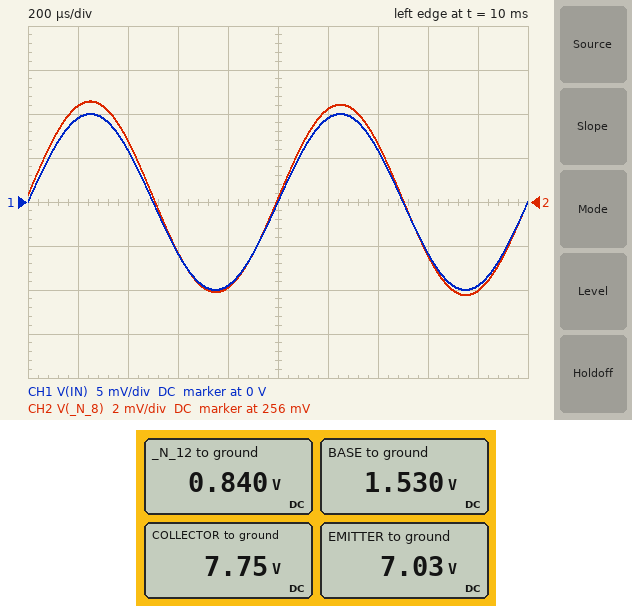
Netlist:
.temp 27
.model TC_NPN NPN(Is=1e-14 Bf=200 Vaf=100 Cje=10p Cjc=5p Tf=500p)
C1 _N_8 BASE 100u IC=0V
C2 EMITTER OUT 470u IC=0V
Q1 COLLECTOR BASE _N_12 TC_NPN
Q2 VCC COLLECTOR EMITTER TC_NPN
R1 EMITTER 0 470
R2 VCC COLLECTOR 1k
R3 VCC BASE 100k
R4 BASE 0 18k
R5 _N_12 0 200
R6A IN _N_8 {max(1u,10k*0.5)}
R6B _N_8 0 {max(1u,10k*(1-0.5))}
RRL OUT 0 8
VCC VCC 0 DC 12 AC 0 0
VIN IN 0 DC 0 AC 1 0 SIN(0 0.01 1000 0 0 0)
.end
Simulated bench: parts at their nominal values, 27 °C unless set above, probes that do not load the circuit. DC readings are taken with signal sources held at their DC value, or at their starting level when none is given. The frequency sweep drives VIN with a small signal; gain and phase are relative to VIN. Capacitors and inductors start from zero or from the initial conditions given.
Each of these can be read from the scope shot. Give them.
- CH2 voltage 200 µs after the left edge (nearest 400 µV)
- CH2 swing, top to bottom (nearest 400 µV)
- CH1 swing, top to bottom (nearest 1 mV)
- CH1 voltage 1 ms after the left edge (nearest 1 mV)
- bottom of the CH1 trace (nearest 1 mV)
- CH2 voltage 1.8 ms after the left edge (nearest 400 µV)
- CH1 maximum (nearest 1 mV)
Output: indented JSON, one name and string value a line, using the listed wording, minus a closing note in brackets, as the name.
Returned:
{
  "CH2 voltage 200 µs after the left edge": "260.4 mV",
  "CH2 swing, top to bottom": "8.8 mV",
  "CH1 swing, top to bottom": "20 mV",
  "CH1 voltage 1 ms after the left edge": "0 V",
  "bottom of the CH1 trace": "-10 mV",
  "CH2 voltage 1.8 ms after the left edge": "252.0 mV",
  "CH1 maximum": "10 mV"
}
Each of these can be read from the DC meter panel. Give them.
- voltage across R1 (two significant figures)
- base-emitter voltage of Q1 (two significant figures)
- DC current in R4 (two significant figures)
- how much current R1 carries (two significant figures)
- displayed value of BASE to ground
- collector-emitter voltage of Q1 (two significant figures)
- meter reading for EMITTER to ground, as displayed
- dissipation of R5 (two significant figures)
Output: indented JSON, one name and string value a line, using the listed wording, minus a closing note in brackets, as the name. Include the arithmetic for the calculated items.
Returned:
{
  "voltage across R1": "7.03 V = 7.0 V",
  "base-emitter voltage of Q1": "1.53 V - 840 mV = 690 mV",
  "DC current in R4": "(1.53 V) / 18 kΩ = 85 µA",
  "how much current R1 carries": "(7.03 V) / 470 Ω = 15 mA",
  "displayed value of BASE to ground": "1.530 V",
  "collector-emitter voltage of Q1": "7.75 V - 840 mV = 6.9 V",
  "meter reading for EMITTER to ground, as displayed": "7.03 V",
  "dissipation of R5": "(840 mV)^2 / 200 Ω = 3.5 mW"
}
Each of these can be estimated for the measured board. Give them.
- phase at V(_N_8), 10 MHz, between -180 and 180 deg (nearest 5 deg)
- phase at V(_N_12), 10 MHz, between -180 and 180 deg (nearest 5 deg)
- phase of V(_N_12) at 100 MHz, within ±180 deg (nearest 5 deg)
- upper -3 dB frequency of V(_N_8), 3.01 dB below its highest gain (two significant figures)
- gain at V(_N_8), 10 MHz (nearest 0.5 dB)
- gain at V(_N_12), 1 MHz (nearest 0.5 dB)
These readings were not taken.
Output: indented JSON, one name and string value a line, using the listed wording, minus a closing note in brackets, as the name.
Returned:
{
  "phase at V(_N_8), 10 MHz, between -180 and 180 deg": "-30 deg",
  "phase at V(_N_12), 10 MHz, between -180 and 180 deg": "-30 deg",
  "phase of V(_N_12) at 100 MHz, within ±180 deg": "-65 deg",
  "upper -3 dB frequency of V(_N_8), 3.01 dB below its highest gain": "6.1 MHz",
  "gain at V(_N_8), 10 MHz": "-11.5 dB",
  "gain at V(_N_12), 1 MHz": "-8.5 dB"
}
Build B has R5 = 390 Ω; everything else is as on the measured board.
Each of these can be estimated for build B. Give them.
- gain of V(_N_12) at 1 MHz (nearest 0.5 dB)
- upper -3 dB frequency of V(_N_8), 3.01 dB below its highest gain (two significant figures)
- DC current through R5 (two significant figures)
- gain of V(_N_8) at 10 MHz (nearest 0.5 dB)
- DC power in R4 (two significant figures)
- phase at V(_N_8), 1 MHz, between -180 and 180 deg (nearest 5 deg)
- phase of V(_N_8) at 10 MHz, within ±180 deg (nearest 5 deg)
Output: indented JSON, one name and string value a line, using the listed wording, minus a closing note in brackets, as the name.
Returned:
{
  "gain of V(_N_12) at 1 MHz": "-8.0 dB",
  "upper -3 dB frequency of V(_N_8), 3.01 dB below its highest gain": "14 MHz",
  "DC current through R5": "2.5 mA",
  "gain of V(_N_8) at 10 MHz": "-10.0 dB",
  "DC power in R4": "150 µW",
  "phase at V(_N_8), 1 MHz, between -180 and 180 deg": "-5 deg",
  "phase of V(_N_8) at 10 MHz, within ±180 deg": "-25 deg"
}
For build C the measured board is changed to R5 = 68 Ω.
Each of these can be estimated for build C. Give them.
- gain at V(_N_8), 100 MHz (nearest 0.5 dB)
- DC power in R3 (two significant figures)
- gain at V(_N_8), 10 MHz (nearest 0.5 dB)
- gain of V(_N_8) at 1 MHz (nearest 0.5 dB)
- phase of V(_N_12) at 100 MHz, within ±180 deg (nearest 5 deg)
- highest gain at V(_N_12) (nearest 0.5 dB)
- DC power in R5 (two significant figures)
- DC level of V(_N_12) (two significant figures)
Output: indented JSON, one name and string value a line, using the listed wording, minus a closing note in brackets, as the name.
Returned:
{
  "gain at V(_N_8), 100 MHz": "-30.5 dB",
  "DC power in R3": "1.2 mW",
  "gain at V(_N_8), 10 MHz": "-17.5 dB",
  "gain of V(_N_8) at 1 MHz": "-10.0 dB",
  "phase of V(_N_12) at 100 MHz, within ±180 deg": "-65 deg",
  "highest gain at V(_N_12)": "-9.0 dB",
  "DC power in R5": "4.3 mW",
  "DC level of V(_N_12)": "540 mV"
}
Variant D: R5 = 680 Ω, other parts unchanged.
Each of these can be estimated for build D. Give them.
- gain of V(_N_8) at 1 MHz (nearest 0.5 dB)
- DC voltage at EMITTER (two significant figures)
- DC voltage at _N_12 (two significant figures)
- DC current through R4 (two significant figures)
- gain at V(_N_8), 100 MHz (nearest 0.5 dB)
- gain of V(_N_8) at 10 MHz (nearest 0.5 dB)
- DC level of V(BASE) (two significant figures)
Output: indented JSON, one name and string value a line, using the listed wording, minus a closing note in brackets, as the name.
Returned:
{
  "gain of V(_N_8) at 1 MHz": "-7.5 dB",
  "DC voltage at EMITTER": "9.6 V",
  "DC voltage at _N_12": "1.1 V",
  "DC current through R4": "96 µA",
  "gain at V(_N_8), 100 MHz": "-20.0 dB",
  "gain of V(_N_8) at 10 MHz": "-9.0 dB",
  "DC level of V(BASE)": "1.7 V"
}
